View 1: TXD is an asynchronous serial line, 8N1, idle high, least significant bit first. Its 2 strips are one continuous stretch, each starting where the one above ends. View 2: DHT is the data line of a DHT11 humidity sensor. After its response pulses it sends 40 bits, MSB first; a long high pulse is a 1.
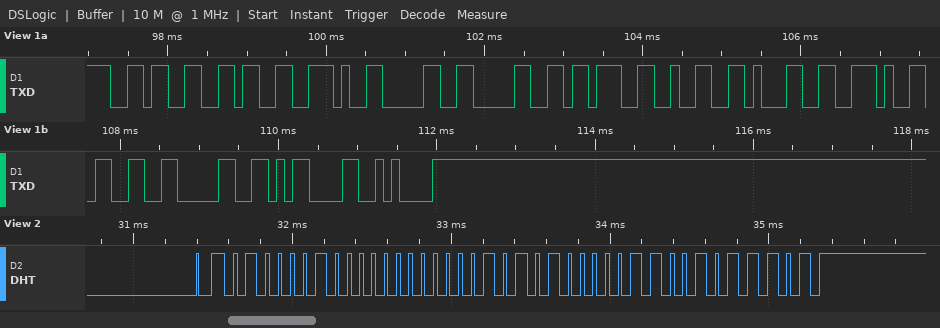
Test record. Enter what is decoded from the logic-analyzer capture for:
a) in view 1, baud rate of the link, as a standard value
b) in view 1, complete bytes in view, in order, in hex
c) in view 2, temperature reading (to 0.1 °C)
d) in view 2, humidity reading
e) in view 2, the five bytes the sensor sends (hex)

9600 baud
36 36 2E 30 30 3B 32 31 2E 33 30 0D 0A
21.6 °C
66 %
42 00 15 06 5D
